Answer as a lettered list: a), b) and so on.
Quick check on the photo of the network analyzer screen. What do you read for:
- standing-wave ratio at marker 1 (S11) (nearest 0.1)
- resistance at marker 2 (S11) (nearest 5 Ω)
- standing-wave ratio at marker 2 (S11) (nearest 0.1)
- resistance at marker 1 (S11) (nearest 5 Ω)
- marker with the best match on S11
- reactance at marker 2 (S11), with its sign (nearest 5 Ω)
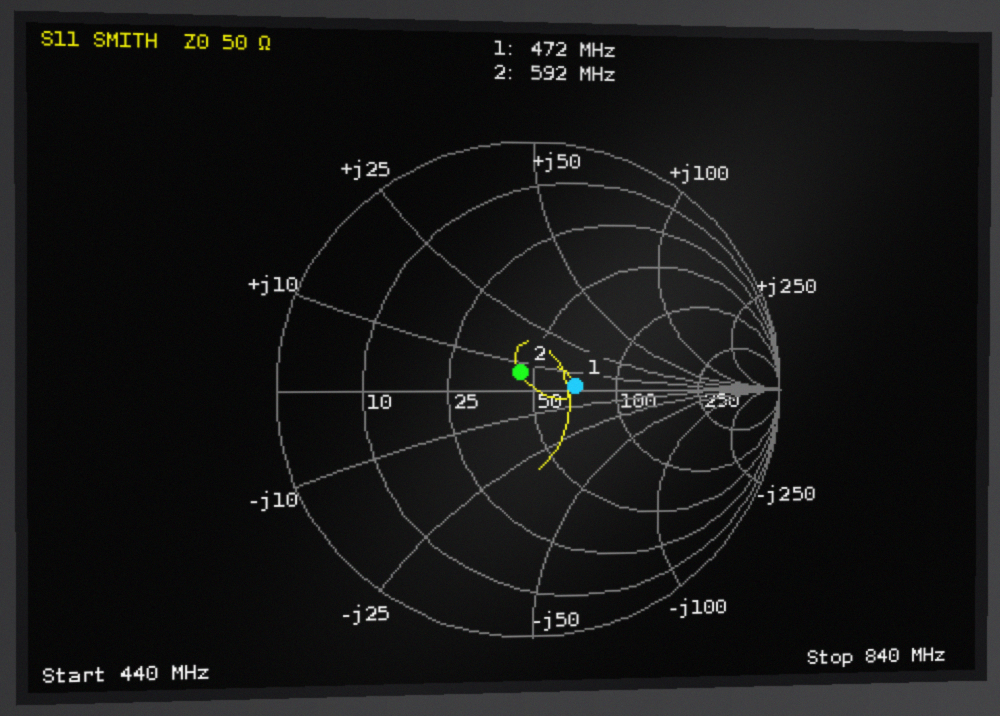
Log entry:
a) 1.4
b) 45 Ω
c) 1.2
d) 70 Ω
e) marker 2
f) +5 Ω
